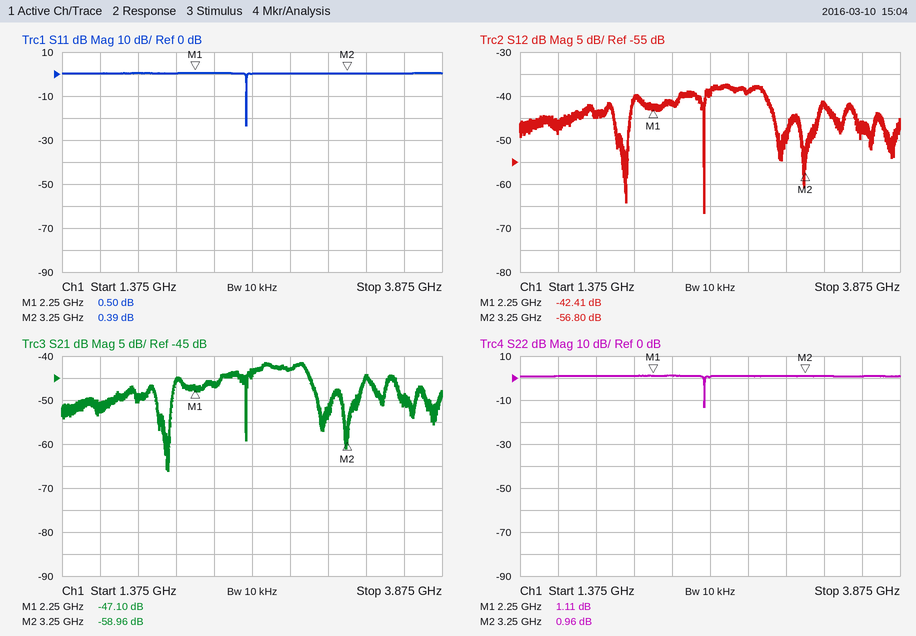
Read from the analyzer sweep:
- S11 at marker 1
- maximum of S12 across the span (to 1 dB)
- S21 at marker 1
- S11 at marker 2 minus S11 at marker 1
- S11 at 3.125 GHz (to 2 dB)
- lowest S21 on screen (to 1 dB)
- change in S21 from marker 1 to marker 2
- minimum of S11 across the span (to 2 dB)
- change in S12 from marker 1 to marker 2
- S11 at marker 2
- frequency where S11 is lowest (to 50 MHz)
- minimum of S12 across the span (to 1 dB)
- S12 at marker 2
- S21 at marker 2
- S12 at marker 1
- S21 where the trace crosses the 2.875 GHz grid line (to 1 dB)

0.50 dB
-37 dB
-47.10 dB
-0.11 dB
0 dB
-66 dB
-11.86 dB
-24 dB
-14.39 dB
0.39 dB
2.60 GHz
-67 dB
-56.80 dB
-58.96 dB
-42.41 dB
-43 dB
